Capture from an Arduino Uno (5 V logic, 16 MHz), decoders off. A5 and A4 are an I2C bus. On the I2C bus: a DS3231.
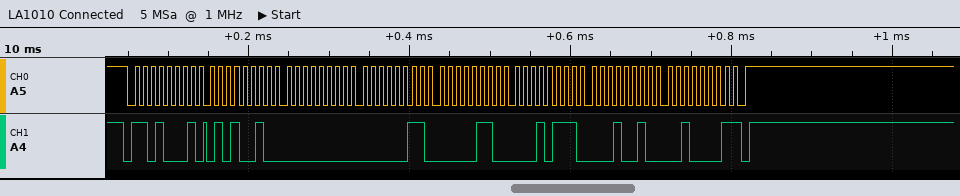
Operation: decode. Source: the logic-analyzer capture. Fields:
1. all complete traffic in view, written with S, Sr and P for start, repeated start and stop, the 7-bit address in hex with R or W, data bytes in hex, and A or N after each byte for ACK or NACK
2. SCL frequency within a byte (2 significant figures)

S 68R A 52 A 00 A 03 A 06 A 17 A 12 A 21 N P
100 kHz
